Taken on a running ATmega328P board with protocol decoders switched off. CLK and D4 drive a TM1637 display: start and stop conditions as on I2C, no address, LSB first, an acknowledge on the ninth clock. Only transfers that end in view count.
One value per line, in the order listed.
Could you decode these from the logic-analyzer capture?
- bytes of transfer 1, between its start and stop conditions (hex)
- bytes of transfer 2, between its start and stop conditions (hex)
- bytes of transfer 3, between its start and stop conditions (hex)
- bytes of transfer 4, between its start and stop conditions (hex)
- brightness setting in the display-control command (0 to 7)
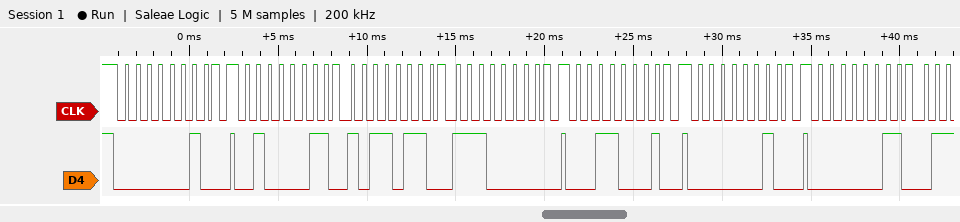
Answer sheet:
40
C2 6D 07
8C
40
4
